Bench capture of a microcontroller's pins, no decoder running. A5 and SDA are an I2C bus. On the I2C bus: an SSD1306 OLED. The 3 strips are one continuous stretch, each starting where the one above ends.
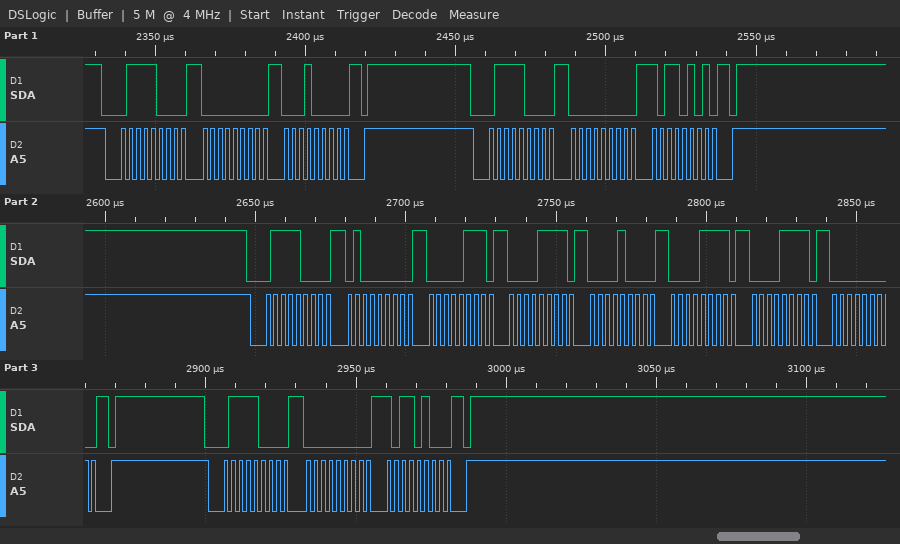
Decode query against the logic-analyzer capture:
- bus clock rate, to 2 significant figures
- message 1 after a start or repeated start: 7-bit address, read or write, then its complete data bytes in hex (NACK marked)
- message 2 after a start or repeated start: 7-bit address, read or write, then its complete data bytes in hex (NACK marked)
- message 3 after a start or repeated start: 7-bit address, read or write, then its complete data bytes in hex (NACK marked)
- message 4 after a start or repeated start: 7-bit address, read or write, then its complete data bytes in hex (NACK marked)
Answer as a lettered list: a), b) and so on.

a) 400 kHz
b) 0x3C write: 00 10
c) 0x3C write: 00 B5
d) 0x3C write: 40 07 0F 08 0F 0F 00
e) 0x3C write: 00 B4
